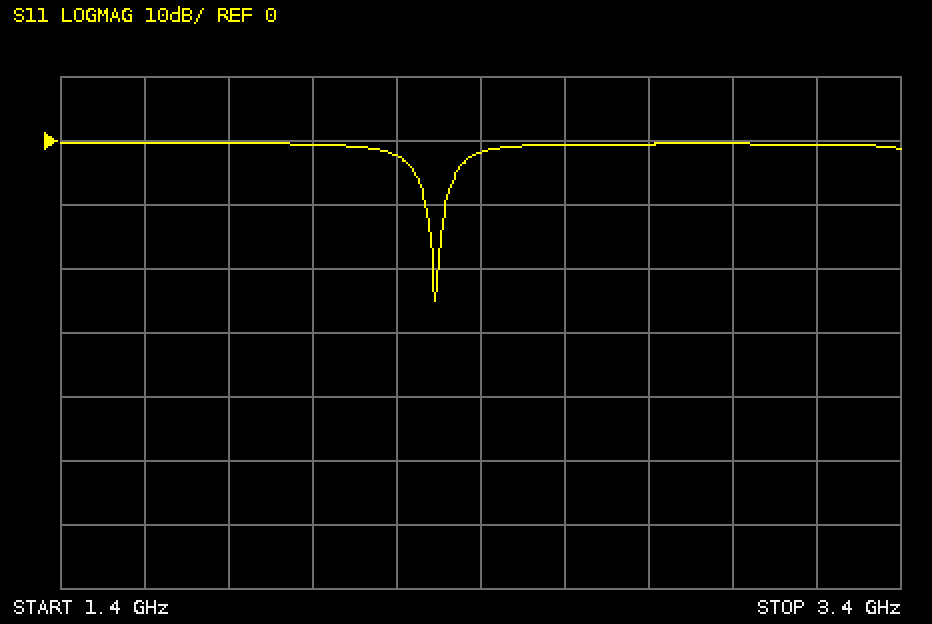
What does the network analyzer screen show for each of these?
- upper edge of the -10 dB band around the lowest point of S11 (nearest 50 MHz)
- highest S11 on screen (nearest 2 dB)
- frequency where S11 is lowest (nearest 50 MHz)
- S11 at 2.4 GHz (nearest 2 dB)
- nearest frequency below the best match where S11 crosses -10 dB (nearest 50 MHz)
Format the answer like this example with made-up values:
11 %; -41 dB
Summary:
2.30 GHz; 0 dB; 2.30 GHz; -2 dB; 2.25 GHz
